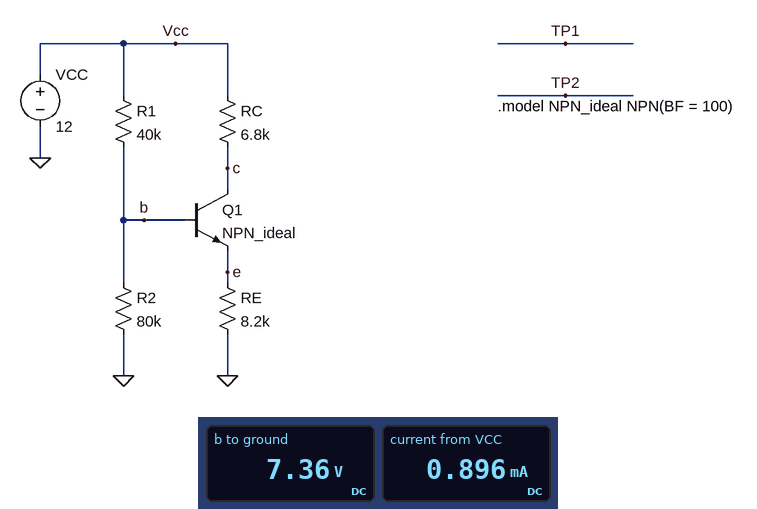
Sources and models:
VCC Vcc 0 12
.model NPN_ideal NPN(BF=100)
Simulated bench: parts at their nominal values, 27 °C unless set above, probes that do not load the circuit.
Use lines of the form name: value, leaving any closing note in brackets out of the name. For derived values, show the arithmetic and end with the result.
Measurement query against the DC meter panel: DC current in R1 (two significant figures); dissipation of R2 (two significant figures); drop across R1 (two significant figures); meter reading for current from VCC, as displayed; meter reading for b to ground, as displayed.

DC current in R1: (12 V - 7.36 V) / 40 kΩ = 120 µA
dissipation of R2: (7.36 V)^2 / 80 kΩ = 680 µW
drop across R1: 12 V - 7.36 V = 4.6 V
meter reading for current from VCC, as displayed: 0.896 mA
meter reading for b to ground, as displayed: 7.36 V
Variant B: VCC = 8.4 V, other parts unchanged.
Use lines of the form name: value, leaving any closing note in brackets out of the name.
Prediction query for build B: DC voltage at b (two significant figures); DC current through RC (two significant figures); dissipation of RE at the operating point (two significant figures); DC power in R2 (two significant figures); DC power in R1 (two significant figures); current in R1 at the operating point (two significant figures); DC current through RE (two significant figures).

DC voltage at b: 5.3 V
DC current through RC: 550 µA
dissipation of RE at the operating point: 2.5 mW
DC power in R2: 350 µW
DC power in R1: 240 µW
current in R1 at the operating point: 77 µA
DC current through RE: 560 µA
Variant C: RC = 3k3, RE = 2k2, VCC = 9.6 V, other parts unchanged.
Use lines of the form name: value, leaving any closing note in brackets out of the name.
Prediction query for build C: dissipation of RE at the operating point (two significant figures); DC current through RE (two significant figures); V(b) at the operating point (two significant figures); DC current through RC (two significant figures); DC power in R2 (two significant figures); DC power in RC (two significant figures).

dissipation of RE at the operating point: 6.9 mW
DC current through RE: 1.8 mA
V(b) at the operating point: 4.7 V
DC current through RC: 1.7 mA
DC power in R2: 270 µW
DC power in RC: 9.6 mW
